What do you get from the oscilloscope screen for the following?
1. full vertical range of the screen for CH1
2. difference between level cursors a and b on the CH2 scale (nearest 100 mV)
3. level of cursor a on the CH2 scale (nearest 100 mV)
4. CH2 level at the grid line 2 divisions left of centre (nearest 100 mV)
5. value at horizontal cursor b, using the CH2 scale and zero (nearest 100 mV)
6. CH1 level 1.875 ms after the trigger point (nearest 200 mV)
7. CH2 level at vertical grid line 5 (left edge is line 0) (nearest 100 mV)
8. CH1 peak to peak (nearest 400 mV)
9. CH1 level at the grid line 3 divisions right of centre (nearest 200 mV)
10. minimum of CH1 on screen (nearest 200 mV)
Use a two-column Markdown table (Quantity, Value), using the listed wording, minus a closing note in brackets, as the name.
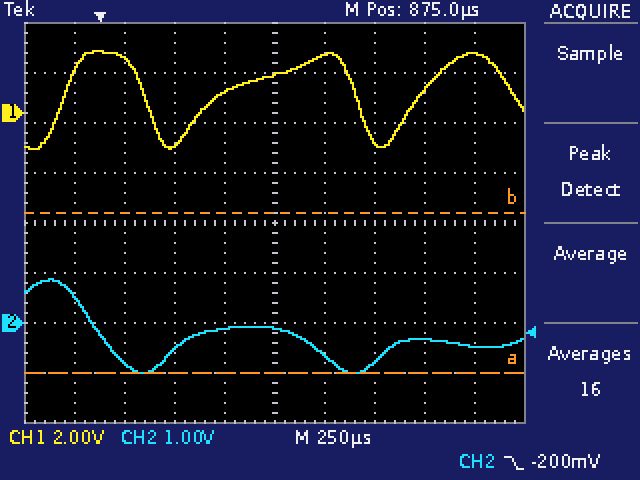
| Quantity | Value |
|---|---|
| full vertical range of the screen for CH1 | 16 V |
| difference between level cursors a and b on the CH2 scale | 3.2 V |
| level of cursor a on the CH2 scale | -1.0 V |
| CH2 level at the grid line 2 divisions left of centre | -500 mV |
| value at horizontal cursor b, using the CH2 scale and zero | 2.2 V |
| CH1 level 1.875 ms after the trigger point | 2.4 V |
| CH2 level at vertical grid line 5 (left edge is line 0) | -100 mV |
| CH1 peak to peak | 4.0 V |
| CH1 level at the grid line 3 divisions right of centre | 1.0 V |
| minimum of CH1 on screen | -1.4 V |
